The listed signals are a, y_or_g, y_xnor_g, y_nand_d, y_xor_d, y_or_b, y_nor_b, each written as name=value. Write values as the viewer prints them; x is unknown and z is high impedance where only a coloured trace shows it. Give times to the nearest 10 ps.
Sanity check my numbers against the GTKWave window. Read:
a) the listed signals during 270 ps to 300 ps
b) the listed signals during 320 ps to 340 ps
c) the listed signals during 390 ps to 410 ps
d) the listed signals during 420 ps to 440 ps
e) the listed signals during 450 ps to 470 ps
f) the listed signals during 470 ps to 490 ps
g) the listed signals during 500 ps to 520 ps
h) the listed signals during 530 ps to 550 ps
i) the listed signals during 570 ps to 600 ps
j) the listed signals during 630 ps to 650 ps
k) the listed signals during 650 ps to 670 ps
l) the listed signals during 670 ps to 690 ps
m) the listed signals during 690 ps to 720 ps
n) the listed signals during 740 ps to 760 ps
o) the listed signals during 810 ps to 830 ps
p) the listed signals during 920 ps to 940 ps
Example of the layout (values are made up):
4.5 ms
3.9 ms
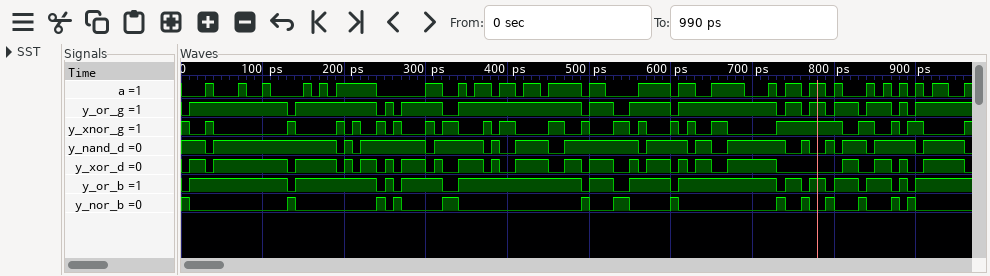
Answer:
a=0, y_or_g=1, y_xnor_g=0, y_nand_d=1, y_xor_d=1, y_or_b=1, y_nor_b=0
a=0, y_or_g=0, y_xnor_g=1, y_nand_d=1, y_xor_d=0, y_or_b=0, y_nor_b=1
a=1, y_or_g=1, y_xnor_g=1, y_nand_d=0, y_xor_d=0, y_or_b=1, y_nor_b=0
a=1, y_or_g=1, y_xnor_g=0, y_nand_d=1, y_xor_d=1, y_or_b=1, y_nor_b=0
a=1, y_or_g=1, y_xnor_g=1, y_nand_d=0, y_xor_d=0, y_or_b=1, y_nor_b=0
a=1, y_or_g=1, y_xnor_g=0, y_nand_d=1, y_xor_d=1, y_or_b=1, y_nor_b=0
a=1, y_or_g=1, y_xnor_g=0, y_nand_d=1, y_xor_d=1, y_or_b=1, y_nor_b=0
a=0, y_or_g=0, y_xnor_g=1, y_nand_d=1, y_xor_d=0, y_or_b=0, y_nor_b=1
a=1, y_or_g=1, y_xnor_g=0, y_nand_d=1, y_xor_d=1, y_or_b=1, y_nor_b=0
a=0, y_or_g=1, y_xnor_g=0, y_nand_d=1, y_xor_d=1, y_or_b=1, y_nor_b=0
a=1, y_or_g=1, y_xnor_g=1, y_nand_d=0, y_xor_d=0, y_or_b=1, y_nor_b=0
a=1, y_or_g=1, y_xnor_g=0, y_nand_d=1, y_xor_d=1, y_or_b=1, y_nor_b=0
a=0, y_or_g=1, y_xnor_g=0, y_nand_d=1, y_xor_d=1, y_or_b=1, y_nor_b=0
a=1, y_or_g=1, y_xnor_g=1, y_nand_d=0, y_xor_d=0, y_or_b=1, y_nor_b=0
a=0, y_or_g=1, y_xnor_g=0, y_nand_d=1, y_xor_d=1, y_or_b=1, y_nor_b=0
a=1, y_or_g=1, y_xnor_g=0, y_nand_d=1, y_xor_d=1, y_or_b=1, y_nor_b=0
